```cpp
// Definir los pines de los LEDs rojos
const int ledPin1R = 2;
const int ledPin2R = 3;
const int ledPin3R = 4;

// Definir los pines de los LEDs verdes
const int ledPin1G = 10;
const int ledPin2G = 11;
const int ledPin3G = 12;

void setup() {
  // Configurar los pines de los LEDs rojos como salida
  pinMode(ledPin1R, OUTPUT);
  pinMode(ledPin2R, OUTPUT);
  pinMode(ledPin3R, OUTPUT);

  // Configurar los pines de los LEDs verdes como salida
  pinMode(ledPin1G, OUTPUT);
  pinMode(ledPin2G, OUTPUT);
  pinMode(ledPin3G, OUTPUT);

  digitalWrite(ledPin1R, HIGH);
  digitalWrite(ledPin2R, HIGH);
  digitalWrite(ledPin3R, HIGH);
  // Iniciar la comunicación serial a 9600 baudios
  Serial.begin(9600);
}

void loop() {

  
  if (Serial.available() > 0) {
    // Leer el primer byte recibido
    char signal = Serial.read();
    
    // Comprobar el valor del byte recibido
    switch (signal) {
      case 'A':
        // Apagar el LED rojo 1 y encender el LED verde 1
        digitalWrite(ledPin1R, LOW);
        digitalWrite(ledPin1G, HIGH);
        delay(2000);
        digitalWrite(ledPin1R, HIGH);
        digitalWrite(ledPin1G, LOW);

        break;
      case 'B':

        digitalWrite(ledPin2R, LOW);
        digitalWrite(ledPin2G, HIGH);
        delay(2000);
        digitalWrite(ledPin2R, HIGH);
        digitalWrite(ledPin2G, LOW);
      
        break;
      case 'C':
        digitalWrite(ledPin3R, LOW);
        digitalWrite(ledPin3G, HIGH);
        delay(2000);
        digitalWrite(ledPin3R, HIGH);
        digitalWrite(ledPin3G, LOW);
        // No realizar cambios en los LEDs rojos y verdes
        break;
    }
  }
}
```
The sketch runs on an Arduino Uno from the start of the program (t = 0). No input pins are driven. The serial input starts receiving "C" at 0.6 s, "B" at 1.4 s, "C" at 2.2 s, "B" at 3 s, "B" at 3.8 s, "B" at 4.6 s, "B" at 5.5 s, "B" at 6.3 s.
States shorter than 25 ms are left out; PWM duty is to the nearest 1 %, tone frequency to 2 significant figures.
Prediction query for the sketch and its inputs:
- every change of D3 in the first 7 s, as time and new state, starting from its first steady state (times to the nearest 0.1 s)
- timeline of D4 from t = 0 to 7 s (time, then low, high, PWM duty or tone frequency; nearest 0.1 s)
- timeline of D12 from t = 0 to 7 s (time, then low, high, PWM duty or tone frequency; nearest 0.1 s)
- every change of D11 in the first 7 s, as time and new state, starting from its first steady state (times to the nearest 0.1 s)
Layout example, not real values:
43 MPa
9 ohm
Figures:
0 s high; 2.6 s low; 4.6 s high; 6.6 s low
0 s high; 0.6 s low; 2.6 s high; 4.6 s low; 6.6 s high
0 s low; 0.6 s high; 2.6 s low; 4.6 s high; 6.6 s low
0 s low; 2.6 s high; 4.6 s low; 6.6 s high
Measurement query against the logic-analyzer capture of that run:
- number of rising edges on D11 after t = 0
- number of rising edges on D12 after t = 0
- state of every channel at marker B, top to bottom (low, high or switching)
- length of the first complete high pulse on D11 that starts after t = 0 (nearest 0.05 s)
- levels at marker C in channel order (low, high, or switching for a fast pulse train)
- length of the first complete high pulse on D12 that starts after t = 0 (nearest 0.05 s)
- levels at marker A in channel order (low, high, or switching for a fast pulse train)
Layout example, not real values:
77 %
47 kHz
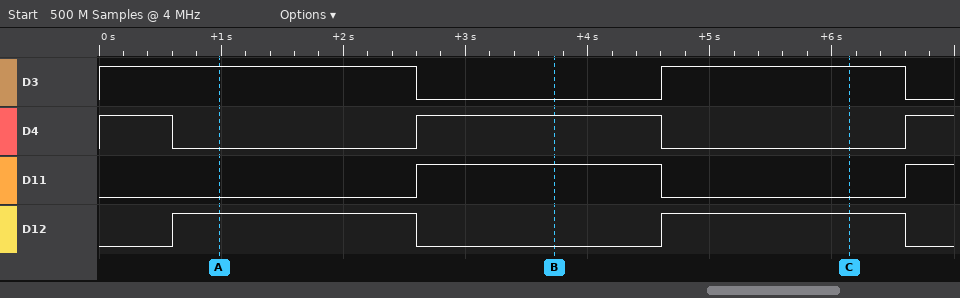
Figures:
2
2
D3 low, D4 high, D11 high, D12 low
2.00 s
D3 high, D4 low, D11 low, D12 high
2.00 s
D3 high, D4 low, D11 low, D12 high
